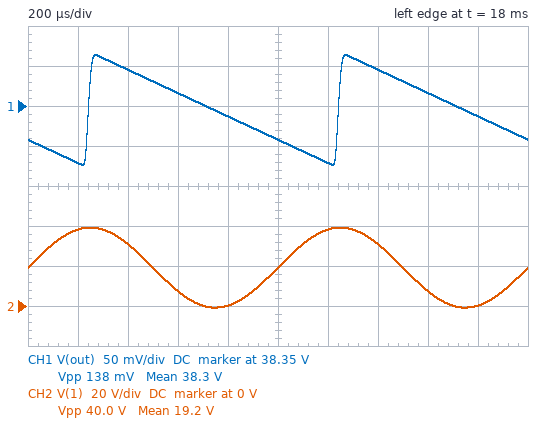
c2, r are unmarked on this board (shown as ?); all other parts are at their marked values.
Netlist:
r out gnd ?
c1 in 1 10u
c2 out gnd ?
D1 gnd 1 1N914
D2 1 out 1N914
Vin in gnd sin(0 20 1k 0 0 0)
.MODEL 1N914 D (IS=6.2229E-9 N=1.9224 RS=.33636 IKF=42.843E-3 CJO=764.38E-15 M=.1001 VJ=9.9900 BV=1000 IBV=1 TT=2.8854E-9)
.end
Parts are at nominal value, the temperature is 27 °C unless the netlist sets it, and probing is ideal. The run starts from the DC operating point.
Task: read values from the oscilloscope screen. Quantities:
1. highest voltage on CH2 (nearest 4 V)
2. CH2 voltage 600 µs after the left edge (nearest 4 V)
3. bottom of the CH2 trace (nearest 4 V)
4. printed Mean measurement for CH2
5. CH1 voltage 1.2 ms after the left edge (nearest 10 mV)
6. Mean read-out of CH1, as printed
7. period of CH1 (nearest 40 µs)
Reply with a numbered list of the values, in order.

1. 40 V
2. 8 V
3. 0 V
4. 19.2 V
5. 38.28 V
6. 38.3 V
7. 1.00 ms
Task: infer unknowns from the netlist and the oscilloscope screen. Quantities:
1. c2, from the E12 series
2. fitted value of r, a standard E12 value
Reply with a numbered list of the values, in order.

1. 4.7 µF
2. 56 kΩ
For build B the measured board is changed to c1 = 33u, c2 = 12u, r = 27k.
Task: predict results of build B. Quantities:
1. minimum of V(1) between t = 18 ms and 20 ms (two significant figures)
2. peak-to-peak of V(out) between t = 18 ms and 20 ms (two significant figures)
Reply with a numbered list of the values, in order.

1. -870 mV
2. 110 mV
